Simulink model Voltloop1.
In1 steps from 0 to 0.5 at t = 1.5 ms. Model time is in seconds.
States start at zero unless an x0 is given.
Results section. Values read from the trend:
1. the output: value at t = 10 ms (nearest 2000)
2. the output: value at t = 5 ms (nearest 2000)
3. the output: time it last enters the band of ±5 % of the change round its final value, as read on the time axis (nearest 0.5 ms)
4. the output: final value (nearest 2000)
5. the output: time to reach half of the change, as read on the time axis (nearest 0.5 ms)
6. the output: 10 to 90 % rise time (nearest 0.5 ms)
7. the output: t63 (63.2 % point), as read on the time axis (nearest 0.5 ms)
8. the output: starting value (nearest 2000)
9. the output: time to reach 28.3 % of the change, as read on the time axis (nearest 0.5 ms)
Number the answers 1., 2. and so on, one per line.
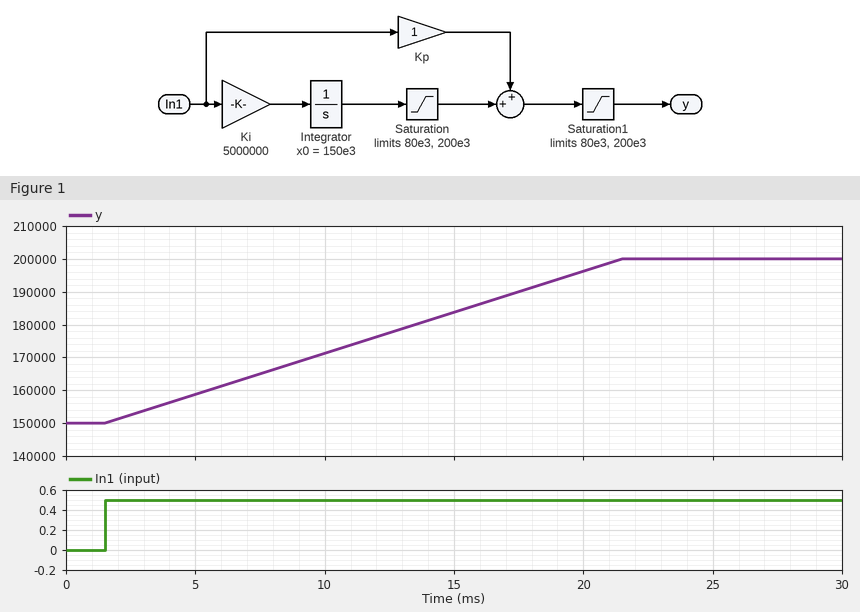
1. 172000
2. 158000
3. 20.5 ms
4. 200000
5. 11.5 ms
6. 16.0 ms
7. 14.0 ms
8. 150000
9. 7.0 ms
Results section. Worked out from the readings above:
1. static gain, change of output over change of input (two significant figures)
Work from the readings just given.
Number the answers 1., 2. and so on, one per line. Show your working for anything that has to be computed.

1. (200000 - 150000) / (0.5 - 0) = 100000
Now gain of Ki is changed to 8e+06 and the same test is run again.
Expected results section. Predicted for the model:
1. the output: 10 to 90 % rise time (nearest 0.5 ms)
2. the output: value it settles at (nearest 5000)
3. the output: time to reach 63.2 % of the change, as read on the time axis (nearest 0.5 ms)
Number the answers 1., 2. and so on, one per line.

1. 10.0 ms
2. 200000
3. 9.5 ms
